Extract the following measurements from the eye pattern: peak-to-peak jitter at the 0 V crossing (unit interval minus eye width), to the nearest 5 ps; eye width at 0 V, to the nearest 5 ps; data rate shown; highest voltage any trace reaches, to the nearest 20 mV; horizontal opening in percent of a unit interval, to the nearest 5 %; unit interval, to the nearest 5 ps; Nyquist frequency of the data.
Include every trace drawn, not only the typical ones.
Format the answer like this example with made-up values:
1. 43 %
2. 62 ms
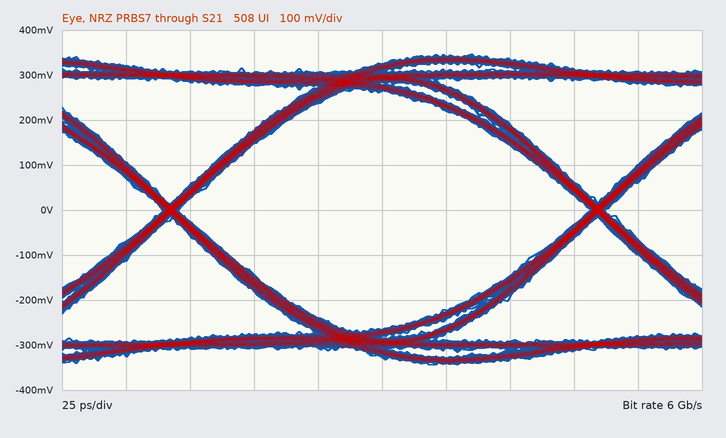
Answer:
1. 5 ps
2. 160 ps
3. 6 Gb/s
4. 340 mV
5. 95 %
6. 165 ps
7. 3 GHz
